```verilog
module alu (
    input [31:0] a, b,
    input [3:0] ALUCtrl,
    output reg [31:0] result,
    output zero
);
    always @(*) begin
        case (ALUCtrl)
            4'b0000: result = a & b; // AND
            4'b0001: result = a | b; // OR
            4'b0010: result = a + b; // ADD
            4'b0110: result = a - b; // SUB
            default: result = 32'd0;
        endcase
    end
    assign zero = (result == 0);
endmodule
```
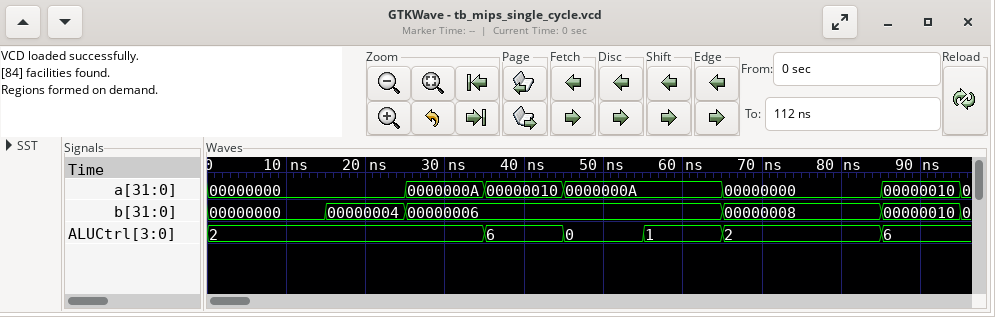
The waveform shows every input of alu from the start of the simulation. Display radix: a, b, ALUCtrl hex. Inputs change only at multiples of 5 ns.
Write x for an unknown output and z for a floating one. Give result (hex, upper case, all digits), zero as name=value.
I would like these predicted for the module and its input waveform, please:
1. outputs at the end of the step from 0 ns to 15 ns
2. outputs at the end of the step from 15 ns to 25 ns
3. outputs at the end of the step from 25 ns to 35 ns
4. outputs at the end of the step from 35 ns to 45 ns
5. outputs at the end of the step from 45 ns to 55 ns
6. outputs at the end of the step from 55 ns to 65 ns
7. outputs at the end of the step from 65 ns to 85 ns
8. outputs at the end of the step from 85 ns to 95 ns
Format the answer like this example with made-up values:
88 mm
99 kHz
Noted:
result=00000000, zero=1
result=00000004, zero=0
result=00000010, zero=0
result=0000000A, zero=0
result=00000002, zero=0
result=0000000E, zero=0
result=00000008, zero=0
result=00000000, zero=1
